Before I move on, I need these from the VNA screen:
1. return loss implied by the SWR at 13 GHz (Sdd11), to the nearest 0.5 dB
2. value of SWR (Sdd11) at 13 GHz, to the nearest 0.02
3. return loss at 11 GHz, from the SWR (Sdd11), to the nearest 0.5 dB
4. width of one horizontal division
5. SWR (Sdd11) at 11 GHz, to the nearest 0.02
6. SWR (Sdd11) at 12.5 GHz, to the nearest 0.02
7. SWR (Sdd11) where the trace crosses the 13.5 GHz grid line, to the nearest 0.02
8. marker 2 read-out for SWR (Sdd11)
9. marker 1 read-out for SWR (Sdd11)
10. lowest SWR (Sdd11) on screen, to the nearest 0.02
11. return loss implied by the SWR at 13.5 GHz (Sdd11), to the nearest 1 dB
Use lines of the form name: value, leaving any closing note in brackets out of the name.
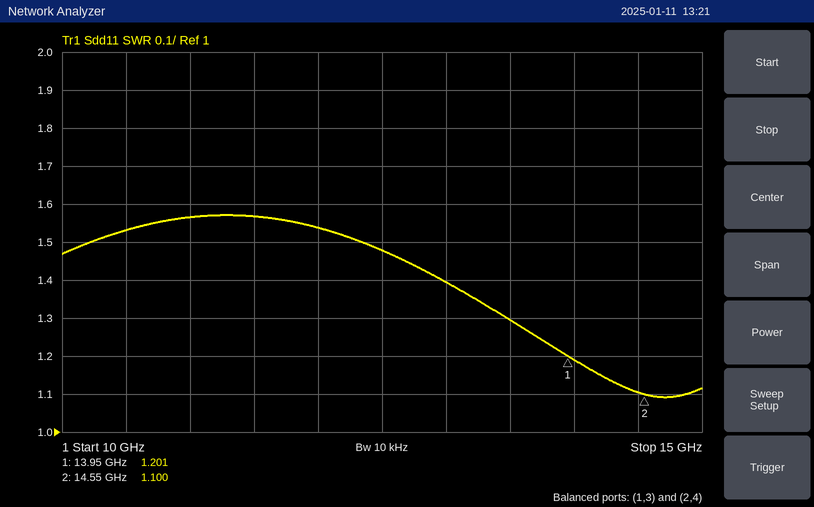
return loss implied by the SWR at 13 GHz (Sdd11), to the nearest 0.5 dB: 15.5 dB
value of SWR (Sdd11) at 13 GHz, to the nearest 0.02: 1.40
return loss at 11 GHz, from the SWR (Sdd11), to the nearest 0.5 dB: 13.0 dB
width of one horizontal division: 500 MHz
SWR (Sdd11) at 11 GHz, to the nearest 0.02: 1.56
SWR (Sdd11) at 12.5 GHz, to the nearest 0.02: 1.48
SWR (Sdd11) where the trace crosses the 13.5 GHz grid line, to the nearest 0.02: 1.30
marker 2 read-out for SWR: 1.100
marker 1 read-out for SWR: 1.201
lowest SWR (Sdd11) on screen, to the nearest 0.02: 1.10
return loss implied by the SWR at 13.5 GHz (Sdd11), to the nearest 1 dB: 18 dB
